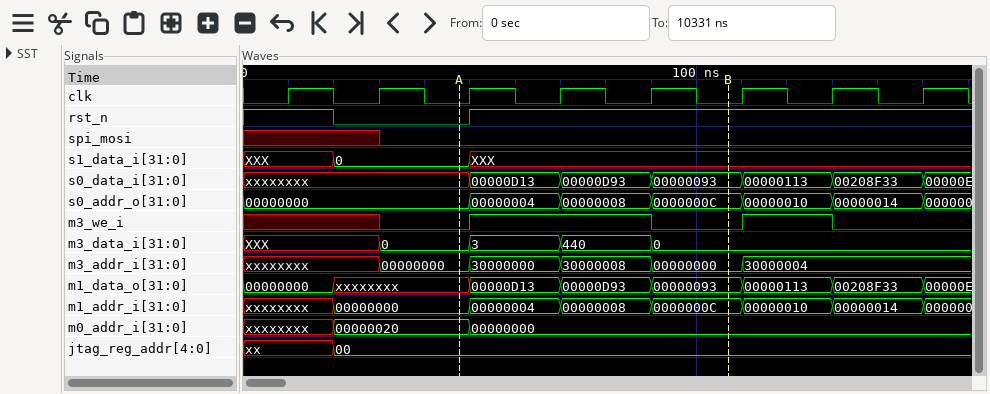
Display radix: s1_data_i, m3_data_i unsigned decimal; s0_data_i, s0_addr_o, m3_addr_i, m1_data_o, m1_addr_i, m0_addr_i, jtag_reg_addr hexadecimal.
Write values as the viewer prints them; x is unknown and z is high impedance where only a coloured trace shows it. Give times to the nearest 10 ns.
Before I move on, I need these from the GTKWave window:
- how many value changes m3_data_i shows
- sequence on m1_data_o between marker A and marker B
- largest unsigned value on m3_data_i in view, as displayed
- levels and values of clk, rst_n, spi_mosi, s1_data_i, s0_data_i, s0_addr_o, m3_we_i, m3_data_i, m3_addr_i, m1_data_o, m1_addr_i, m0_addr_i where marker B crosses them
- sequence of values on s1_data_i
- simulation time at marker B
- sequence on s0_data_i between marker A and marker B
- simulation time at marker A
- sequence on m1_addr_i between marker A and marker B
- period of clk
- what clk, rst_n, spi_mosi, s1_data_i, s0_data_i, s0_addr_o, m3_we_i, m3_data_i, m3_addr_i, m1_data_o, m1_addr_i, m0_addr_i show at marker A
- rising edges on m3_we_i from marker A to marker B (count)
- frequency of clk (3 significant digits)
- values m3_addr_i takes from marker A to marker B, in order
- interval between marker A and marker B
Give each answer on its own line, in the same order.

4
xxxxxxxx, 00000D13, 00000D93, 00000093
440
clk=0, rst_n=1, spi_mosi=0, s1_data_i=XXX, s0_data_i=00000093, s0_addr_o=0000000C, m3_we_i=0, m3_data_i=0, m3_addr_i=00000000, m1_data_o=00000093, m1_addr_i=0000000C, m0_addr_i=00000000
XXX, 0, XXX
110 ns
xxxxxxxx, 00000D13, 00000D93, 00000093
50 ns
00000000, 00000004, 00000008, 0000000C
20 ns
clk=0, rst_n=0, spi_mosi=0, s1_data_i=0, s0_data_i=xxxxxxxx, s0_addr_o=00000000, m3_we_i=0, m3_data_i=0, m3_addr_i=00000000, m1_data_o=xxxxxxxx, m1_addr_i=00000000, m0_addr_i=00000020
1
50.0 MHz
00000000, 30000000, 30000008, 00000000
60 ns
